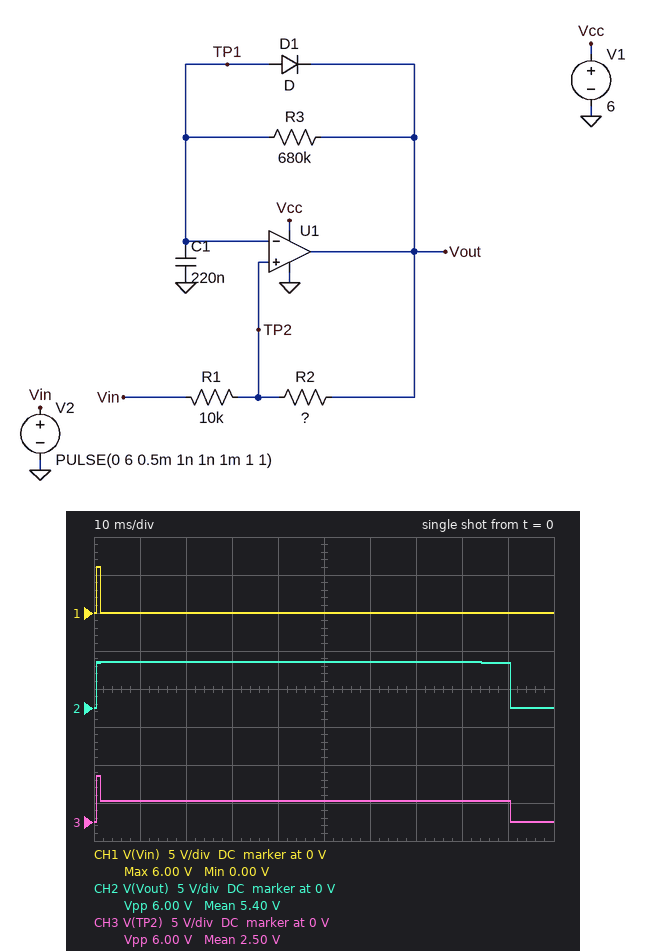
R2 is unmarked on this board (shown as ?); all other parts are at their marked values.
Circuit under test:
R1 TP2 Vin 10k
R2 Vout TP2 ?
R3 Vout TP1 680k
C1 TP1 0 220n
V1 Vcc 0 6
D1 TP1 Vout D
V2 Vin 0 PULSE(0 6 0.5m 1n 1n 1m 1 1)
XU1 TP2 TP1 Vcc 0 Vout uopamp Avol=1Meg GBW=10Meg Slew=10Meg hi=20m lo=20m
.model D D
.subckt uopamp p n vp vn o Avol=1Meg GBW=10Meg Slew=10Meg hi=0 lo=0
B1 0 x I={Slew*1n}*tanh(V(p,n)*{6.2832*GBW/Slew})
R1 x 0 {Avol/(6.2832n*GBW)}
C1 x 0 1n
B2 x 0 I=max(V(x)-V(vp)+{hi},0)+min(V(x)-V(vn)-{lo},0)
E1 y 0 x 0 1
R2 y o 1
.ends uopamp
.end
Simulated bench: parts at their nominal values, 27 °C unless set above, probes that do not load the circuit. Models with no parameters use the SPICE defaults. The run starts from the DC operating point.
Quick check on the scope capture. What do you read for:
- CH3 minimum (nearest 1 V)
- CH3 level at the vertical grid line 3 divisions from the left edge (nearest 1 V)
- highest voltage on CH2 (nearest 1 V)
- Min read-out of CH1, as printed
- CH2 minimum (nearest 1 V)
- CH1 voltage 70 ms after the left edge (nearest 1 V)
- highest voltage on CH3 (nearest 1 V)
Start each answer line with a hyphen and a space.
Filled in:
- 0 V
- 3 V
- 6 V
- 0.00 V
- 0 V
- 0 V
- 6 V
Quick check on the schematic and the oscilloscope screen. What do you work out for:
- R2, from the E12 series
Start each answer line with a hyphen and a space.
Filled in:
- 12 kΩ
